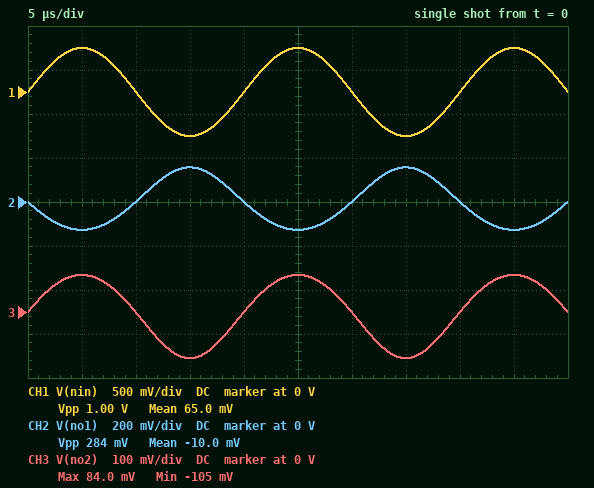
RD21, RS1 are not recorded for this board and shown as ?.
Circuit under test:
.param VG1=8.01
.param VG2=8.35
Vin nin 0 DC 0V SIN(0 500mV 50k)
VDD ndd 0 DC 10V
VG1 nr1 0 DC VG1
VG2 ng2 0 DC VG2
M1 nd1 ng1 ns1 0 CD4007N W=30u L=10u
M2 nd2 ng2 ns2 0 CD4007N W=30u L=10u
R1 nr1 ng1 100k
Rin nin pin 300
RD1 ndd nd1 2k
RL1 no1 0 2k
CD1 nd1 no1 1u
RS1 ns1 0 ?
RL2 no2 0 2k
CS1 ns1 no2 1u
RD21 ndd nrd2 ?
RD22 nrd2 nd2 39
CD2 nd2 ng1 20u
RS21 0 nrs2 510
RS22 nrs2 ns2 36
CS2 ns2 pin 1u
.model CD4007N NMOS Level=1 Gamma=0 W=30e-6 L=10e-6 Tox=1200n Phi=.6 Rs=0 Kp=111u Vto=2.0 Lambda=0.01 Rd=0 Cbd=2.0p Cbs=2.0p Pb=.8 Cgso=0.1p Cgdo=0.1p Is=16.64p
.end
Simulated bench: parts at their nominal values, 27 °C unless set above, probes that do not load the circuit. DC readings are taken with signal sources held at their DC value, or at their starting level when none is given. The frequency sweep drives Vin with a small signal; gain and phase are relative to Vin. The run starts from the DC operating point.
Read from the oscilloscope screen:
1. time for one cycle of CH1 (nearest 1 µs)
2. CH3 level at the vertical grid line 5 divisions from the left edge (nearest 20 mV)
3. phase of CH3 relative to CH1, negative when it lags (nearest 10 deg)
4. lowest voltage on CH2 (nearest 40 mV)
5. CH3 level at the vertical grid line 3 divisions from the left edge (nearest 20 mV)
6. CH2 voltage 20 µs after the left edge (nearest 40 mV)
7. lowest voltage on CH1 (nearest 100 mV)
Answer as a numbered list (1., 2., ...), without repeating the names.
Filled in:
1. 20 µs
2. 80 mV
3. 0 deg
4. -120 mV
5. -100 mV
6. 0 V
7. -500 mV
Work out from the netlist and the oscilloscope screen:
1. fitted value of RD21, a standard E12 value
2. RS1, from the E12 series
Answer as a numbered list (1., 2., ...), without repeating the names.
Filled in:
1. 680 Ω
2. 1 kΩ
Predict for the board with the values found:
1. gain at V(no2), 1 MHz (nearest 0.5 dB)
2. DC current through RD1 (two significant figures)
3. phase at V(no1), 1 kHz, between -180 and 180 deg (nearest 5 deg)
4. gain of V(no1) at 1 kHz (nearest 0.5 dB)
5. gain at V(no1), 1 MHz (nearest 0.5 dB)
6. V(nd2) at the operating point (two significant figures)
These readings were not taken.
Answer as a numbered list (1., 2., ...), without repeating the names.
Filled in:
1. -14.5 dB
2. 2.3 mA
3. -160 deg
4. -11.5 dB
5. -11.0 dB
6. 7.5 V
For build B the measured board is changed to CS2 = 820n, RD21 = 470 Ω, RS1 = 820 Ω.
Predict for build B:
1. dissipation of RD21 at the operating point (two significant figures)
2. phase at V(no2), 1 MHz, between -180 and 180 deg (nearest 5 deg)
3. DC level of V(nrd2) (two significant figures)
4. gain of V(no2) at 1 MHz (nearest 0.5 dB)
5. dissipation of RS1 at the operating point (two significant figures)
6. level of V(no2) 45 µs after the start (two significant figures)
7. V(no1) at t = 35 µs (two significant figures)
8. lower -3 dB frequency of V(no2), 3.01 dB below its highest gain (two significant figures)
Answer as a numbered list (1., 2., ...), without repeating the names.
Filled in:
1. 5.7 mW
2. 0 deg
3. 8.4 V
4. -19.5 dB
5. 5.1 mW
6. 49 mV
7. 100 mV
8. 340 Hz
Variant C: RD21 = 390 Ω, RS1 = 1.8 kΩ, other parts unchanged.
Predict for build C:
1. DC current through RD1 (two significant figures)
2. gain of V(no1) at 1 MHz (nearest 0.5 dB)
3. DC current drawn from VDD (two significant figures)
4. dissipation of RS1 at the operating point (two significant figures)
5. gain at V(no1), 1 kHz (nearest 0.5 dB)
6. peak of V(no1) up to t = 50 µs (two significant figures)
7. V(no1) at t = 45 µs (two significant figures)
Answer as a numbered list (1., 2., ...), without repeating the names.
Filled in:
1. 1.6 mA
2. -15.0 dB
3. 5.1 mA
4. 4.8 mW
5. -15.5 dB
6. 89 mV
7. -85 mV
